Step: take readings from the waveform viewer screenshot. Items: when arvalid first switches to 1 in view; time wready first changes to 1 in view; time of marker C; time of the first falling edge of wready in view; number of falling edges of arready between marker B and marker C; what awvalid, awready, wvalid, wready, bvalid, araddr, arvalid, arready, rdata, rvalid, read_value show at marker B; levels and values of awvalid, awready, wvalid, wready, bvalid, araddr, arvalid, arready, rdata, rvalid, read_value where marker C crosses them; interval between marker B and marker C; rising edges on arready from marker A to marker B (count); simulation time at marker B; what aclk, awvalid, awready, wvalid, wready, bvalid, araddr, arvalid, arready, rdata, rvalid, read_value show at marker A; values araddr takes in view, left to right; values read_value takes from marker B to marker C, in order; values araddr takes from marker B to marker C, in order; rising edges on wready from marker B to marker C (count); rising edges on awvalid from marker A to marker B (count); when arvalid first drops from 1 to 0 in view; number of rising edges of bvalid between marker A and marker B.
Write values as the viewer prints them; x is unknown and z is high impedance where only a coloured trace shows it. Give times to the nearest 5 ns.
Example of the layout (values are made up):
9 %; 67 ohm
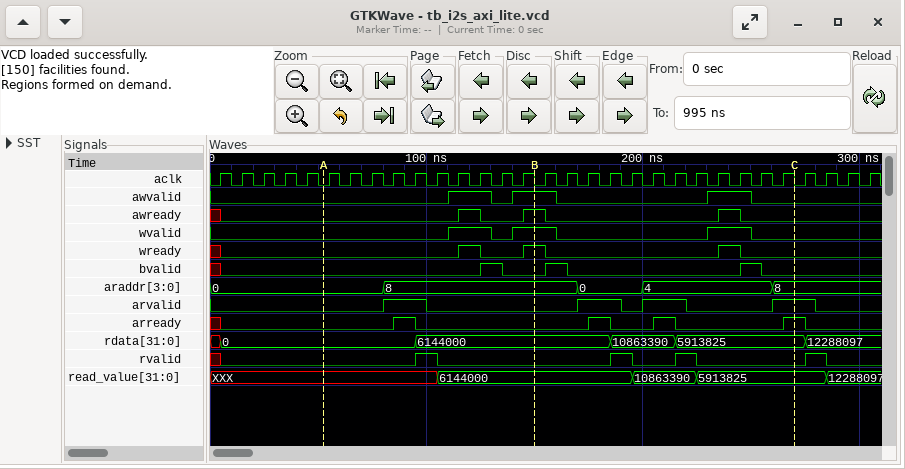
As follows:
80 ns; 115 ns; 270 ns; 125 ns; 2; awvalid=1, awready=1, wvalid=1, wready=1, bvalid=0, araddr=8, arvalid=0, arready=0, rdata=6144000, rvalid=0, read_value=6144000; awvalid=0, awready=0, wvalid=0, wready=0, bvalid=0, araddr=8, arvalid=1, arready=1, rdata=5913825, rvalid=0, read_value=5913825; 120 ns; 1; 150 ns; aclk=0, awvalid=0, awready=0, wvalid=0, wready=0, bvalid=0, araddr=0, arvalid=0, arready=0, rdata=0, rvalid=0, read_value=XXX; 0, 8, 0, 4, 8; 6144000, 10863390, 5913825; 8, 0, 4, 8; 1; 2; 100 ns; 1
